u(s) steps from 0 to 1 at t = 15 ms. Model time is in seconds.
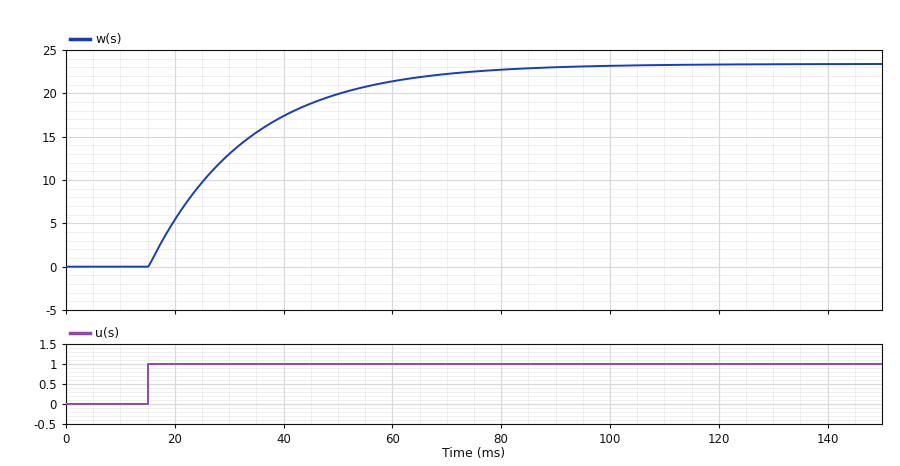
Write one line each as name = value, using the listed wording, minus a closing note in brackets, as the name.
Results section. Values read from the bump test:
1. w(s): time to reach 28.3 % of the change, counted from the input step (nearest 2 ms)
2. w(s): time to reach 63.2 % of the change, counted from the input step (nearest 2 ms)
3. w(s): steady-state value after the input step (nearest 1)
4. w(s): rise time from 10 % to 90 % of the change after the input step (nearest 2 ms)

w(s): time to reach 28.3 % of the change, counted from the input step = 6 ms
w(s): time to reach 63.2 % of the change, counted from the input step = 18 ms
w(s): steady-state value after the input step = 23
w(s): rise time from 10 % to 90 % of the change after the input step = 40 ms
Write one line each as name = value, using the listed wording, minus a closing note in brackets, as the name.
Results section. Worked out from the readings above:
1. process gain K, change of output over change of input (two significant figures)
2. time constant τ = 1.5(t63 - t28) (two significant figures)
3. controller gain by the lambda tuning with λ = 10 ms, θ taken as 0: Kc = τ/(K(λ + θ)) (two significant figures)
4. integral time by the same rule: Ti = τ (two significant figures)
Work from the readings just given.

process gain K, change of output over change of input = 23
time constant τ = 1.5(t63 - t28) = 18 ms
controller gain by the lambda tuning with λ = 10 ms, θ taken as 0: Kc = τ/(K(λ + θ)) = 0.078
integral time by the same rule: Ti = τ = 18 ms
